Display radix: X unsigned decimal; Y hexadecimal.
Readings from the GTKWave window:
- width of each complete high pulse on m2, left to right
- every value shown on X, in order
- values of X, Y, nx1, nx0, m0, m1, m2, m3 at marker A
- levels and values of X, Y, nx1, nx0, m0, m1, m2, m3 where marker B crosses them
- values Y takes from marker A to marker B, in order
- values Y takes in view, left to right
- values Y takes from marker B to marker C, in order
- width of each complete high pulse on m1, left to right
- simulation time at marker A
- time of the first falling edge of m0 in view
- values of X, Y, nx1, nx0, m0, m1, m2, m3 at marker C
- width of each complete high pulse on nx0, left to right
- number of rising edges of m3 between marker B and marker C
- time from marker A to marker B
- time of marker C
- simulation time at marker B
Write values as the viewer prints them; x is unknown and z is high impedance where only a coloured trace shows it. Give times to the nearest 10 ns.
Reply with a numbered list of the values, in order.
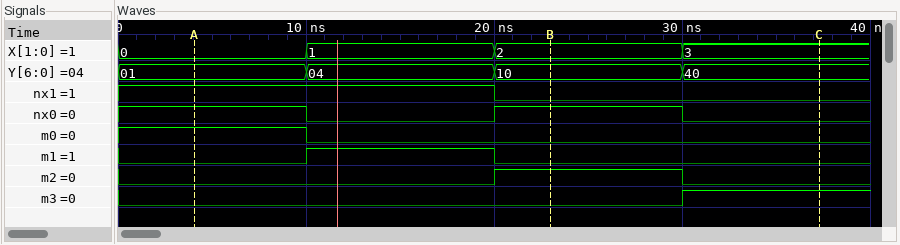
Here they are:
1. 10 ns
2. 0, 1, 2, 3
3. X=0, Y=01, nx1=1, nx0=1, m0=1, m1=0, m2=0, m3=0
4. X=2, Y=10, nx1=0, nx0=1, m0=0, m1=0, m2=1, m3=0
5. 01, 04, 10
6. 01, 04, 10, 40
7. 10, 40
8. 10 ns
9. 0 ns
10. 10 ns
11. X=3, Y=40, nx1=0, nx0=0, m0=0, m1=0, m2=0, m3=1
12. 10 ns
13. 1
14. 20 ns
15. 40 ns
16. 20 ns
